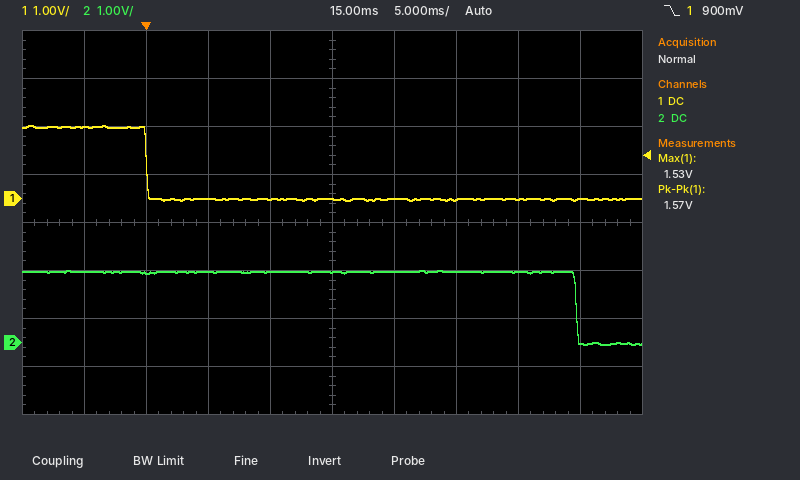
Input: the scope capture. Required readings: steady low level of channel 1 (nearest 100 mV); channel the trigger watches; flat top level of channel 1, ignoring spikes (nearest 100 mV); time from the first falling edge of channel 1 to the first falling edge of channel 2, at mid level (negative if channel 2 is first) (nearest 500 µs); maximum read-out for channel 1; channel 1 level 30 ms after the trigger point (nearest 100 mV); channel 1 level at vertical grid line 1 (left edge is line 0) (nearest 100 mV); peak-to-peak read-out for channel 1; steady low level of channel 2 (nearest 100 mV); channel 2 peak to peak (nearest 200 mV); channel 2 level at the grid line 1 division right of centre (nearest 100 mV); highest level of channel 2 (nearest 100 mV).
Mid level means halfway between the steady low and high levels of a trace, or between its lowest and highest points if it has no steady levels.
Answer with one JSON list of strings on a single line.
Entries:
["0.0 V", "channel 1", "1.5 V", "+34.5 ms", "1.53 V", "0.0 V", "1.5 V", "1.57 V", "0.0 V", "1.6 V", "1.5 V", "1.5 V"]
